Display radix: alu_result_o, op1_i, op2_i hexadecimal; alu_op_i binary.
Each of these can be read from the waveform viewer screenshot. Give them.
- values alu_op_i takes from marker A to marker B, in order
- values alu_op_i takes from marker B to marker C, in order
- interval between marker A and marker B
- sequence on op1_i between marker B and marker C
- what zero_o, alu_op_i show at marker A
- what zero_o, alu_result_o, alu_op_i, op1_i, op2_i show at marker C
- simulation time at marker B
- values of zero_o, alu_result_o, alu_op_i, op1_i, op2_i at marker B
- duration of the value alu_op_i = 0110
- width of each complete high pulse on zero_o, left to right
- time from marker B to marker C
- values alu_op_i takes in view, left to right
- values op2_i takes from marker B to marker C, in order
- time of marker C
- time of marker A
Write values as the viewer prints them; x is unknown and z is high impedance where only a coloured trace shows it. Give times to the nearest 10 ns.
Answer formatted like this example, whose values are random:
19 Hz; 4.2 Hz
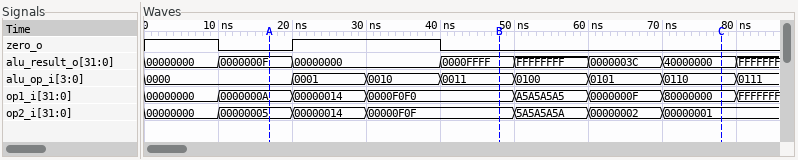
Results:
0000, 0001, 0010, 0011; 0011, 0100, 0101, 0110; 30 ns; 0000F0F0, A5A5A5A5, 0000000F, 80000000; zero_o=0, alu_op_i=0000; zero_o=0, alu_result_o=40000000, alu_op_i=0110, op1_i=80000000, op2_i=00000001; 50 ns; zero_o=0, alu_result_o=0000FFFF, alu_op_i=0011, op1_i=0000F0F0, op2_i=00000F0F; 10 ns; 20 ns; 30 ns; 0000, 0001, 0010, 0011, 0100, 0101, 0110, 0111; 00000F0F, 5A5A5A5A, 00000002, 00000001; 80 ns; 20 ns
